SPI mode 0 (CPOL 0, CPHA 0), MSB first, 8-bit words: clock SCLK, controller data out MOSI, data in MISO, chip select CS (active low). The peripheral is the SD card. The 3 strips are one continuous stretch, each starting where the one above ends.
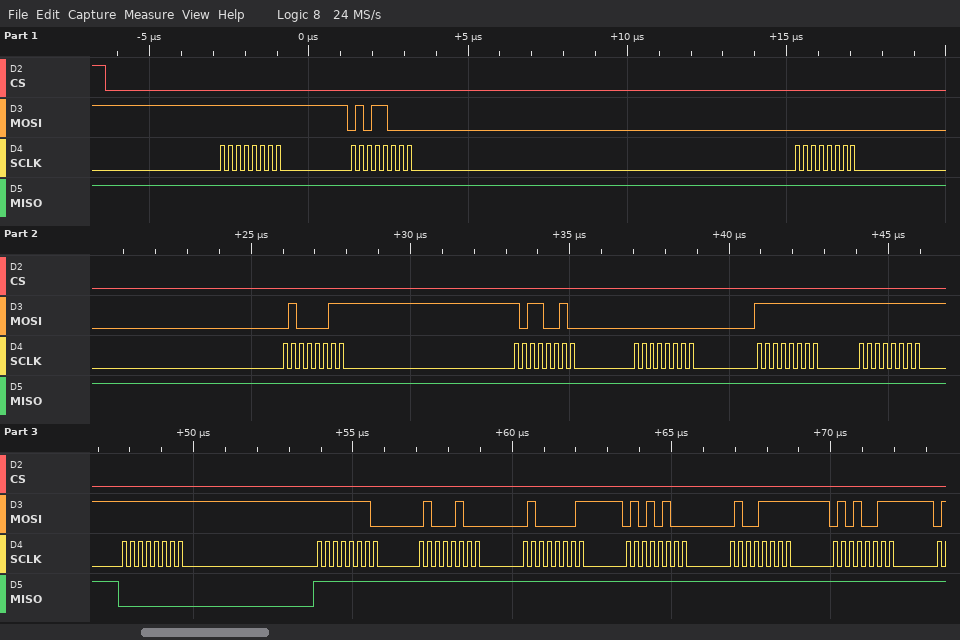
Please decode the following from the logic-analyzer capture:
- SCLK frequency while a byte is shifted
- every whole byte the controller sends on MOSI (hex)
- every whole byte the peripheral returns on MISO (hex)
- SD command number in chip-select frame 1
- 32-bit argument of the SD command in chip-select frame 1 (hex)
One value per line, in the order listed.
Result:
4 MHz
FF 58 00 43 B2 00 FF FF FF FE 44 41 54 4F 53
FF FF FF FF FF FF FF FF 00 FF FF FF FF FF FF
CMD24
0x0043B200
